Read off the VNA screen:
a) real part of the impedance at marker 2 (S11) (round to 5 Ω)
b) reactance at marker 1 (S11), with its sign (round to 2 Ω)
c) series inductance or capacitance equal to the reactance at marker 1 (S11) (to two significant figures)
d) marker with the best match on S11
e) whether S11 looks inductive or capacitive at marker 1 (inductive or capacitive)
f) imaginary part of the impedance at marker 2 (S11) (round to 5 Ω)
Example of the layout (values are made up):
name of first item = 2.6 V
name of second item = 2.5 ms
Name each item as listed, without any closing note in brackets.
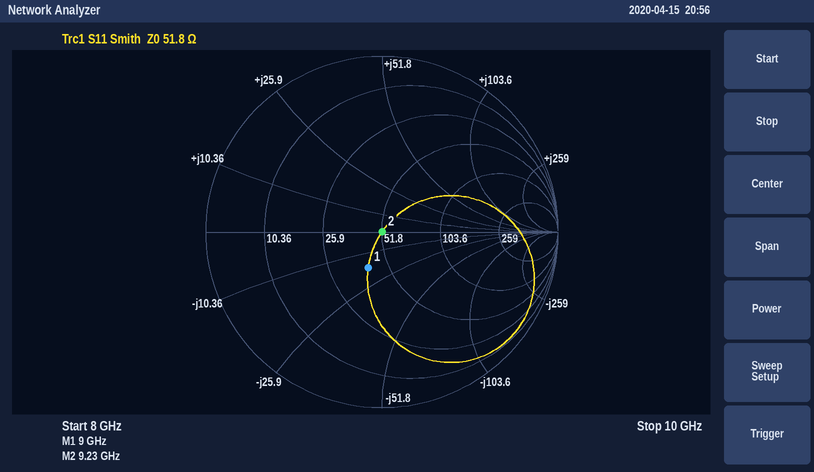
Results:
real part of the impedance at marker 2 (S11) = 50 Ω
reactance at marker 1 (S11), with its sign = -18 Ω
series inductance or capacitance equal to the reactance at marker 1 (S11) = 1.0 pF
marker with the best match on S11 = marker 2
whether S11 looks inductive or capacitive at marker 1 = capacitive
imaginary part of the impedance at marker 2 (S11) = 0 Ω
